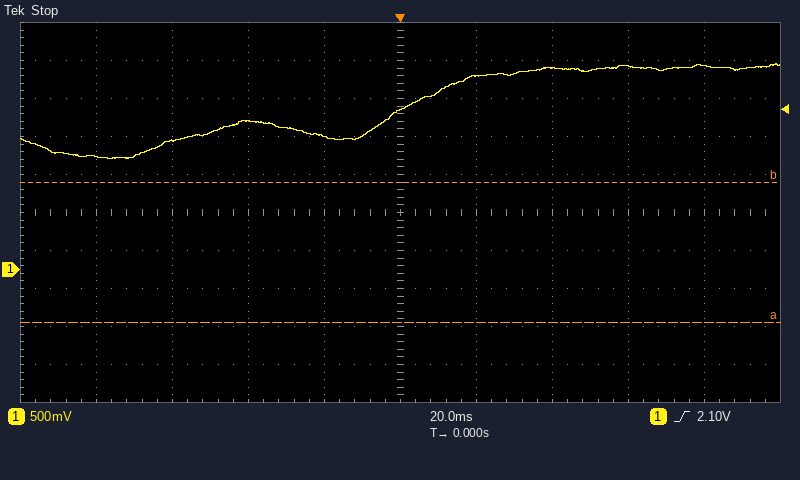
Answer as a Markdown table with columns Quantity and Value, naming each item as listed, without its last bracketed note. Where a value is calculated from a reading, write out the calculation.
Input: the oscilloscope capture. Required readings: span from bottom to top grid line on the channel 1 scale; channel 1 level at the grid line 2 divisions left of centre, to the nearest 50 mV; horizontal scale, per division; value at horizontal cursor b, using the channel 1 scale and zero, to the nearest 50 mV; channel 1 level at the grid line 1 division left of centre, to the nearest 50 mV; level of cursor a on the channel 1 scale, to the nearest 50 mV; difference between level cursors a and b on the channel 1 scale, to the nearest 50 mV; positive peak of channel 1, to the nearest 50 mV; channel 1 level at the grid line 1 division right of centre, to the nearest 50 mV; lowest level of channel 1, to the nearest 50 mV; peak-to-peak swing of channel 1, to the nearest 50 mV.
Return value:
| Quantity | Value |
|---|---|
| span from bottom to top grid line on the channel 1 scale | 5 V |
| channel 1 level at the grid line 2 divisions left of centre, to the nearest 50 mV | 1.95 V |
| horizontal scale, per division | 20 ms |
| value at horizontal cursor b, using the channel 1 scale and zero, to the nearest 50 mV | 1.15 V |
| channel 1 level at the grid line 1 division left of centre, to the nearest 50 mV | 1.75 V |
| level of cursor a on the channel 1 scale, to the nearest 50 mV | -700 mV |
| difference between level cursors a and b on the channel 1 scale, to the nearest 50 mV | 1.85 V |
| positive peak of channel 1, to the nearest 50 mV | 2.70 V |
| channel 1 level at the grid line 1 division right of centre, to the nearest 50 mV | 2.55 V |
| lowest level of channel 1, to the nearest 50 mV | 1.45 V |
| peak-to-peak swing of channel 1, to the nearest 50 mV | 2.70 V − (1.45 V) = 1.25 V |
